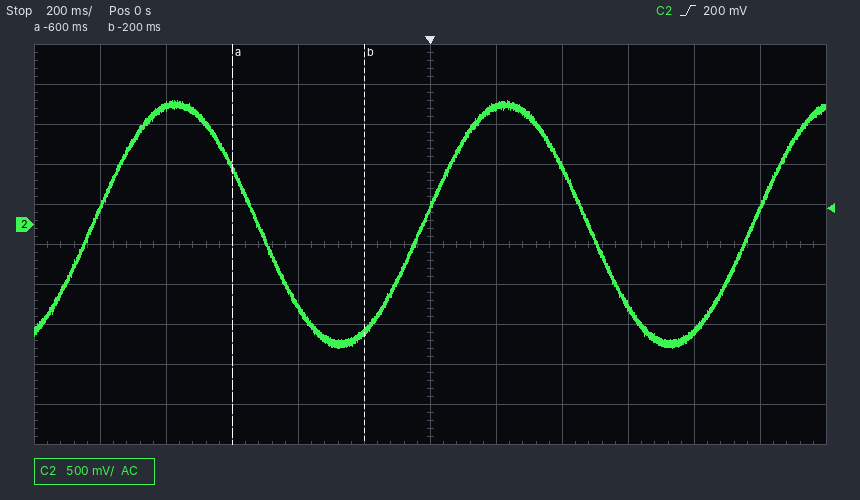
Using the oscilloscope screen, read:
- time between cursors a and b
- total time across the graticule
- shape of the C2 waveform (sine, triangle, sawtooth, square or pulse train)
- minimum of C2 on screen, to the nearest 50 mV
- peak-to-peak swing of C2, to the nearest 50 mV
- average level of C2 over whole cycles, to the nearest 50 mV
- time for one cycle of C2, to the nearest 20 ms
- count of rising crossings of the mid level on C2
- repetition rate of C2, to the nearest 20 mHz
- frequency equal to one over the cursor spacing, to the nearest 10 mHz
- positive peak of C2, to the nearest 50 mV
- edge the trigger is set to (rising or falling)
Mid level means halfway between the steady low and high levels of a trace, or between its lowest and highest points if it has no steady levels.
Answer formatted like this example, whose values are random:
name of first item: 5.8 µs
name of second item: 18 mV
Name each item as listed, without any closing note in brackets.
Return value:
time between cursors a and b: 400 ms
total time across the graticule: 2.4 s
shape of the C2 waveform: sine
minimum of C2 on screen, to the nearest 50 mV: -1.55 V
peak-to-peak swing of C2, to the nearest 50 mV: 3.10 V
average level of C2 over whole cycles, to the nearest 50 mV: 0 mV
time for one cycle of C2, to the nearest 20 ms: 1.00 s
count of rising crossings of the mid level on C2: 3
repetition rate of C2, to the nearest 20 mHz: 1.00 Hz
frequency equal to one over the cursor spacing, to the nearest 10 mHz: 2.50 Hz
positive peak of C2, to the nearest 50 mV: 1.55 V
edge the trigger is set to: rising
